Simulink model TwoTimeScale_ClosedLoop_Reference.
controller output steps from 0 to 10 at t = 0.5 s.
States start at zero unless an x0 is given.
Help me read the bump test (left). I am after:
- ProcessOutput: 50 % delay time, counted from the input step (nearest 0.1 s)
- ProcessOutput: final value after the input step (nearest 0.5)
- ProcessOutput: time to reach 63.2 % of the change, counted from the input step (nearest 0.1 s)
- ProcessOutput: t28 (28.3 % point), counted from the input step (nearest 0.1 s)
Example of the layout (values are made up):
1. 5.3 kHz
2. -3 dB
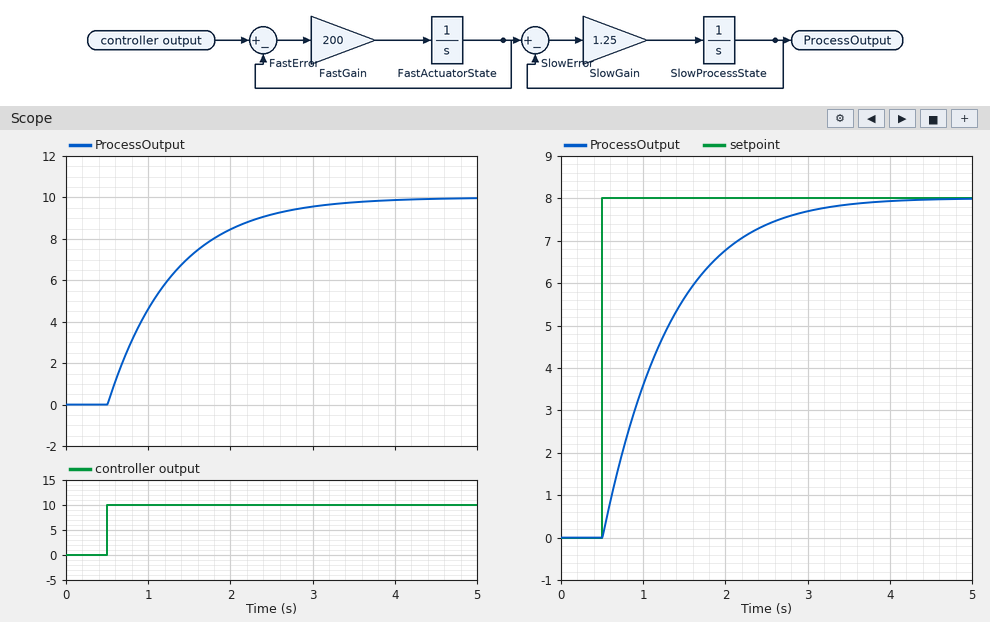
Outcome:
1. 0.6 s
2. 10.0
3. 0.8 s
4. 0.3 s
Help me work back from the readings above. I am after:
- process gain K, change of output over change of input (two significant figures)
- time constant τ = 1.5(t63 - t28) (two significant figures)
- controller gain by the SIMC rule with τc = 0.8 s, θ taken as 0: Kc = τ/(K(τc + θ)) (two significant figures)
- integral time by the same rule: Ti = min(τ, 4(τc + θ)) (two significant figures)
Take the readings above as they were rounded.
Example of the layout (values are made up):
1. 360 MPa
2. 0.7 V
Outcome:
1. 1.0
2. 0.75 s
3. 0.94
4. 0.75 s
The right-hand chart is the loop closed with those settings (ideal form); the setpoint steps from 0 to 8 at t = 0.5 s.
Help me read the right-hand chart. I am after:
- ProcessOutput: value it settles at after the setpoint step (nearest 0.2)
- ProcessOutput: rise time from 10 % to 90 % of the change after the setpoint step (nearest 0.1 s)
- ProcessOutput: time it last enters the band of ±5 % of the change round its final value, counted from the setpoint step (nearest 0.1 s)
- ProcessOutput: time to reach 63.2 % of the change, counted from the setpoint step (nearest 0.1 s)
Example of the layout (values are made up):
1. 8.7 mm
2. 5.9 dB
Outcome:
1. 8.0
2. 1.7 s
3. 2.3 s
4. 0.8 s
